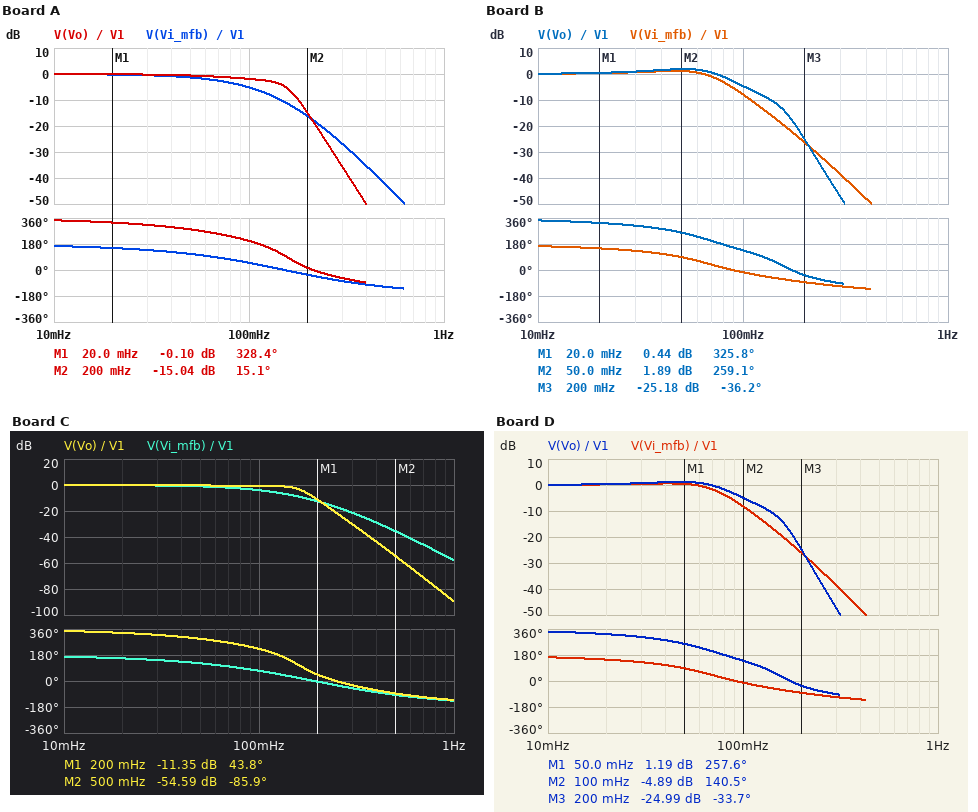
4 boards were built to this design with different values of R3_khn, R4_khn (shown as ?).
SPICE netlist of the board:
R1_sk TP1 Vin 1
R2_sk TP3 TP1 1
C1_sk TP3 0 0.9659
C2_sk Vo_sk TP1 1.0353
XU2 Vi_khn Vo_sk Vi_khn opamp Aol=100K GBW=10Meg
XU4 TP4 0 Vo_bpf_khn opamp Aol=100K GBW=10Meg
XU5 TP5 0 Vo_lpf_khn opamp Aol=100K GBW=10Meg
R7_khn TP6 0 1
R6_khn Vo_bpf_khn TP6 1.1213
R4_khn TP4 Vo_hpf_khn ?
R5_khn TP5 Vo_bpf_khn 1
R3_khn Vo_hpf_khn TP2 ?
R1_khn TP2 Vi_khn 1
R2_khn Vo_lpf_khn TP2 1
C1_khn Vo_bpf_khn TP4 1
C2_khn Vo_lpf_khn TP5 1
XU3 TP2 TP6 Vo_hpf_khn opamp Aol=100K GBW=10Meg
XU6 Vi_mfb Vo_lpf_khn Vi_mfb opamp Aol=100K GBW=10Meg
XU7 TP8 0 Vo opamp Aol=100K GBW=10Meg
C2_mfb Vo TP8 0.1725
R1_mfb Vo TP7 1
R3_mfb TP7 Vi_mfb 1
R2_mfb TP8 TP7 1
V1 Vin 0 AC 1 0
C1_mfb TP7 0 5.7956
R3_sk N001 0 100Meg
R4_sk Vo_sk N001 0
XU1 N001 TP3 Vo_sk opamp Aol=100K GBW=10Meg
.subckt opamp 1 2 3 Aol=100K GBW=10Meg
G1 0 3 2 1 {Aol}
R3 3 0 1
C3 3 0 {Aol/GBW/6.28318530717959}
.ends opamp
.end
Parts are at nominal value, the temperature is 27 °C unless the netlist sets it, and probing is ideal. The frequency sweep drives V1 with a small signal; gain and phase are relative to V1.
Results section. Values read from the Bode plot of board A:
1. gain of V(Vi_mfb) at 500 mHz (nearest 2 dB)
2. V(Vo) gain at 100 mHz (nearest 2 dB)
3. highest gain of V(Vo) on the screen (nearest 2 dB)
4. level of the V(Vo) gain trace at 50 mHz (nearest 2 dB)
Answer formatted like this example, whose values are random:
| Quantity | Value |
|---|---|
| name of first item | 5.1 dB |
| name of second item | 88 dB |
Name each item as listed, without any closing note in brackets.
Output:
| Quantity | Value |
|---|---|
| gain of V(Vi_mfb) at 500 mHz | -42 dB |
| V(Vo) gain at 100 mHz | -2 dB |
| highest gain of V(Vo) on the screen | 0 dB |
| level of the V(Vo) gain trace at 50 mHz | 0 dB |
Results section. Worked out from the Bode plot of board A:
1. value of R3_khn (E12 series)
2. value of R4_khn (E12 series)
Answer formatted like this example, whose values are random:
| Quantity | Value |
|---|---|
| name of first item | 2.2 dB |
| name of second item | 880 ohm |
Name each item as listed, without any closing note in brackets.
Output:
| Quantity | Value |
|---|---|
| value of R3_khn | 0.47 Ω |
| value of R4_khn | 0.56 Ω |
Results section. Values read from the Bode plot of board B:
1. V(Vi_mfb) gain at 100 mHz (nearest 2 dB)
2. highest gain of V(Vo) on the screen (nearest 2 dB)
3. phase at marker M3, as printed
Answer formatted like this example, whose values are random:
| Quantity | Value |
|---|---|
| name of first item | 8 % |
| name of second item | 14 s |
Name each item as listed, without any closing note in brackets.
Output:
| Quantity | Value |
|---|---|
| V(Vi_mfb) gain at 100 mHz | -8 dB |
| highest gain of V(Vo) on the screen | 2 dB |
| phase at marker M3, as printed | -36.2 deg |
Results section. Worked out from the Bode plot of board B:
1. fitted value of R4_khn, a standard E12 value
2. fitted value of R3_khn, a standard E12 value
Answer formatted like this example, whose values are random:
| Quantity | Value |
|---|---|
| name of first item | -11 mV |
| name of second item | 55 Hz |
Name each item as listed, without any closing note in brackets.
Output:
| Quantity | Value |
|---|---|
| fitted value of R4_khn, a standard E12 value | 2.2 Ω |
| fitted value of R3_khn, a standard E12 value | 0.39 Ω |
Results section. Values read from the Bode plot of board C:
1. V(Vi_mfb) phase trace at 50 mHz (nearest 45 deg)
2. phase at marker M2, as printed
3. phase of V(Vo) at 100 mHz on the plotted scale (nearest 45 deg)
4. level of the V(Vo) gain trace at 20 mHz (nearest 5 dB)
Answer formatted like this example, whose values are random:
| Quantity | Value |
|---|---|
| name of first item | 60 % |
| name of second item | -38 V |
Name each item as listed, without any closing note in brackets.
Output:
| Quantity | Value |
|---|---|
| V(Vi_mfb) phase trace at 50 mHz | 135 deg |
| phase at marker M2, as printed | -85.9 deg |
| phase of V(Vo) at 100 mHz on the plotted scale | 225 deg |
| level of the V(Vo) gain trace at 20 mHz | 0 dB |
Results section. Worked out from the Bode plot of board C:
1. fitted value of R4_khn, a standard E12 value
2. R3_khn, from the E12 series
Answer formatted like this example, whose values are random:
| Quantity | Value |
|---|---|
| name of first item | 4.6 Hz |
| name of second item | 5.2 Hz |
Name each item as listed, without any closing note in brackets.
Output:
| Quantity | Value |
|---|---|
| fitted value of R4_khn, a standard E12 value | 0.56 Ω |
| R3_khn, from the E12 series | 1.2 Ω |
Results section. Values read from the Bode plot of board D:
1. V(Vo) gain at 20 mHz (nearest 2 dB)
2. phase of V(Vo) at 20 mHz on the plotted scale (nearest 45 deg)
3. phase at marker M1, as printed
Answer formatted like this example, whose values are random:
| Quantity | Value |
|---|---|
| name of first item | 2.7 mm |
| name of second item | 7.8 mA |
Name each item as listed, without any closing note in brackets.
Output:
| Quantity | Value |
|---|---|
| V(Vo) gain at 20 mHz | 0 dB |
| phase of V(Vo) at 20 mHz on the plotted scale | 315 deg |
| phase at marker M1, as printed | 257.6 deg |
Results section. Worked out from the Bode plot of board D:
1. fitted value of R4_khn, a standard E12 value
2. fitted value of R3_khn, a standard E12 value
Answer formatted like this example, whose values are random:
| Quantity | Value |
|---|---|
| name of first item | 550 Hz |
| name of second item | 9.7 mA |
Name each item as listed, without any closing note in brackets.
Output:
| Quantity | Value |
|---|---|
| fitted value of R4_khn, a standard E12 value | 1.8 Ω |
| fitted value of R3_khn, a standard E12 value | 0.33 Ω |
